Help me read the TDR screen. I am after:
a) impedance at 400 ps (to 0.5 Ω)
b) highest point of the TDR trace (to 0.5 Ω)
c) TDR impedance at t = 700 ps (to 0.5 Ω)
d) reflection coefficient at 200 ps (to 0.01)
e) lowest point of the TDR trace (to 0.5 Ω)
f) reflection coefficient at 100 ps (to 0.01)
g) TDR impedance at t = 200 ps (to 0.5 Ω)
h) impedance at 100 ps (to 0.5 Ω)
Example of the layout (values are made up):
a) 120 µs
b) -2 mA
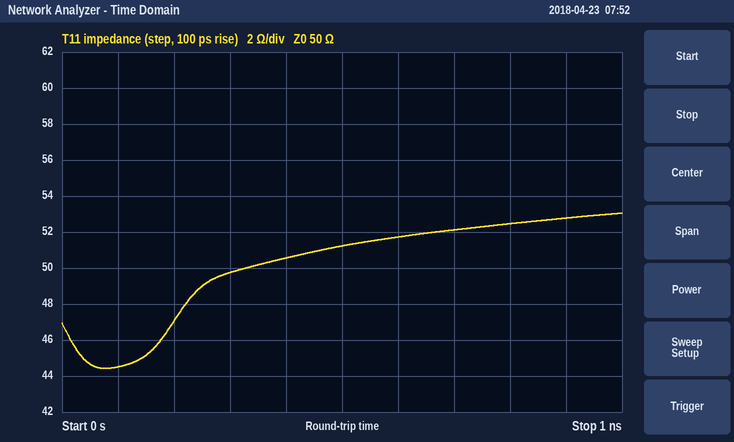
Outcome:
a) 50.5 Ω
b) 53.0 Ω
c) 52.0 Ω
d) -0.03
e) 44.5 Ω
f) -0.06
g) 47.0 Ω
h) 44.5 Ω
